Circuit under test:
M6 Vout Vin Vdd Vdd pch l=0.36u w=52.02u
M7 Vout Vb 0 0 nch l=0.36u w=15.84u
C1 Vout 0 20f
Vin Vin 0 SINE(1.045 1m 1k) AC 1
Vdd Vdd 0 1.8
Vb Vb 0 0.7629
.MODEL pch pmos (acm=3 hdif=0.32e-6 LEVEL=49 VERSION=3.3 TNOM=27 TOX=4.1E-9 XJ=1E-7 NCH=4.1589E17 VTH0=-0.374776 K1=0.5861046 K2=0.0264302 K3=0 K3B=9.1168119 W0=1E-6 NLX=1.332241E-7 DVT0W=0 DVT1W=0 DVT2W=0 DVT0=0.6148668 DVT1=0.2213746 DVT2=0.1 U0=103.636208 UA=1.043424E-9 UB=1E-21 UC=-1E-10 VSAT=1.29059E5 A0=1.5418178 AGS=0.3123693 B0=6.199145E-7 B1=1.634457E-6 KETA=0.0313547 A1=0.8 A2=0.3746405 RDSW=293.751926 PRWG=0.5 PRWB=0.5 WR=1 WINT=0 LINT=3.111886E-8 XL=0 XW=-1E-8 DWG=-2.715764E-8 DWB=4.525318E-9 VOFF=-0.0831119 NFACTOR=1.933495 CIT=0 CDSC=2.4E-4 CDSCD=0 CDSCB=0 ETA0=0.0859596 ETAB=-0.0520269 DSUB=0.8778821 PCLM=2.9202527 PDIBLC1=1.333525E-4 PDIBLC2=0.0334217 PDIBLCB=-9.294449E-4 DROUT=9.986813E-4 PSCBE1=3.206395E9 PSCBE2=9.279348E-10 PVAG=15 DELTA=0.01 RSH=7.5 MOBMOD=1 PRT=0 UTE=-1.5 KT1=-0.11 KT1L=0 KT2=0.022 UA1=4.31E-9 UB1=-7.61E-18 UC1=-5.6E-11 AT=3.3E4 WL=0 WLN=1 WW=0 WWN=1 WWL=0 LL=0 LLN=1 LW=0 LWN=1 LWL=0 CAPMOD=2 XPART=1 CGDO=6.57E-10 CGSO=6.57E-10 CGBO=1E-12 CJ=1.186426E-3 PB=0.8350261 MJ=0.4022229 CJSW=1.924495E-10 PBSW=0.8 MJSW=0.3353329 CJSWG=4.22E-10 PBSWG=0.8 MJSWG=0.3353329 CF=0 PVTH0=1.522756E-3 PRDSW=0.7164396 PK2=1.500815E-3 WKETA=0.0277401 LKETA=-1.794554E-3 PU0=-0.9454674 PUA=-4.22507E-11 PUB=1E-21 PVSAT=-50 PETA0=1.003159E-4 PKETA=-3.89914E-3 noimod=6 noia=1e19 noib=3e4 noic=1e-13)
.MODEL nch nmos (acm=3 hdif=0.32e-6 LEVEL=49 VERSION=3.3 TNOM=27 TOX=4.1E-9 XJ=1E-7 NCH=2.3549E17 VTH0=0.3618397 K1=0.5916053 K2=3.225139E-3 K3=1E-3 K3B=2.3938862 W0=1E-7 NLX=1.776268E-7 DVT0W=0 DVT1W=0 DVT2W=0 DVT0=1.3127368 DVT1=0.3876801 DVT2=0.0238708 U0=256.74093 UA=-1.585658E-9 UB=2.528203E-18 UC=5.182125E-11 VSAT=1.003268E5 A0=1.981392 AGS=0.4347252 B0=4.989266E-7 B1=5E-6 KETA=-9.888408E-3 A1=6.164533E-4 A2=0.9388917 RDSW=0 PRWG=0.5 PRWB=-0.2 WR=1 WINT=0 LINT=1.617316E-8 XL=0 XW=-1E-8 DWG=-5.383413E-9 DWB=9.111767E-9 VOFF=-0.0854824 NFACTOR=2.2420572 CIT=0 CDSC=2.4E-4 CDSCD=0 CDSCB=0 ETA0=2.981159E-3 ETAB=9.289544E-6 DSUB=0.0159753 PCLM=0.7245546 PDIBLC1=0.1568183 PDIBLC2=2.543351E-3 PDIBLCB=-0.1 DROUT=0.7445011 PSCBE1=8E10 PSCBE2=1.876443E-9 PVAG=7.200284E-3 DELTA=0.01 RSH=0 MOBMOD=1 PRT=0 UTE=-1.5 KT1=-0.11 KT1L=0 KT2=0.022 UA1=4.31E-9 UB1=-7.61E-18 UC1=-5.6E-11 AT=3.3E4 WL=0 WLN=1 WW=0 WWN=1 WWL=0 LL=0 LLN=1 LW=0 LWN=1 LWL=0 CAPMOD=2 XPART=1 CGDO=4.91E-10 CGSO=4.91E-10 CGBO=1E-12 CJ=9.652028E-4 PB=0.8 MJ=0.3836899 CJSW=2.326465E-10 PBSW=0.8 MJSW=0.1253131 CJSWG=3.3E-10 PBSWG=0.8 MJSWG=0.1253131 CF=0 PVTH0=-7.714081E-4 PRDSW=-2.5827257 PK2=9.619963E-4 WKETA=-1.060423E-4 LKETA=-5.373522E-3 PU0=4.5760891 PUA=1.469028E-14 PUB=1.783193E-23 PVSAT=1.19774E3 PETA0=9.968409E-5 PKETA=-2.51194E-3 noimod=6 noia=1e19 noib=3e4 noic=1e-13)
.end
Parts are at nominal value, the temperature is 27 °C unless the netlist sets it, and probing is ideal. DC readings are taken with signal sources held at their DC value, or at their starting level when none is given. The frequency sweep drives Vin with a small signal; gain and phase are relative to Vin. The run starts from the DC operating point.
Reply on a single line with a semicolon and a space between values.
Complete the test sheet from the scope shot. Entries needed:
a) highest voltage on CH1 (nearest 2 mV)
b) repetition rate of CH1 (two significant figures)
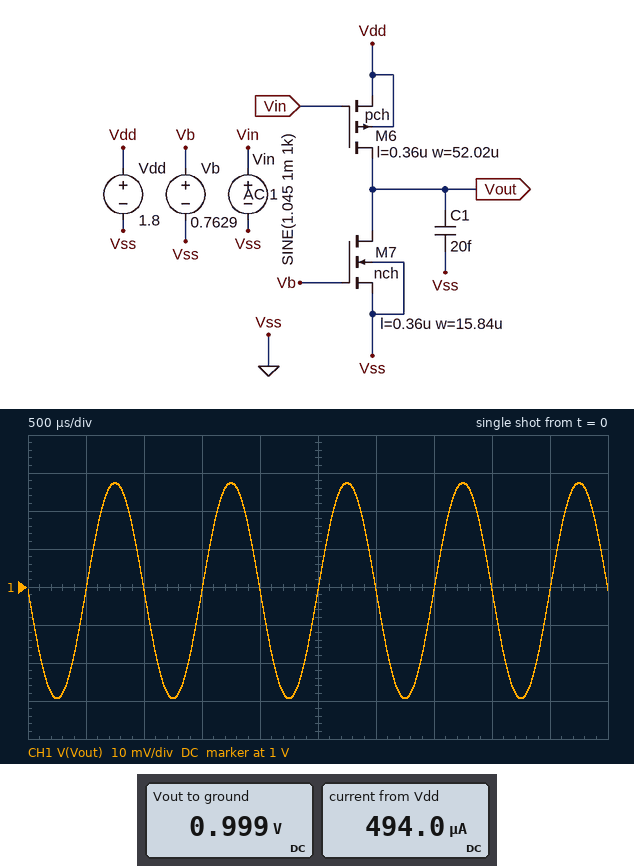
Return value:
1.028 V; 1.0 kHz
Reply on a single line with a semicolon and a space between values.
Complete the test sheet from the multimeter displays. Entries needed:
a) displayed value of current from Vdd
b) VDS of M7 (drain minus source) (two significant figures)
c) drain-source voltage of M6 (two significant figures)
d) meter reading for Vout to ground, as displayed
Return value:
494.0 µA; 1.0 V; -800 mV; 0.999 V
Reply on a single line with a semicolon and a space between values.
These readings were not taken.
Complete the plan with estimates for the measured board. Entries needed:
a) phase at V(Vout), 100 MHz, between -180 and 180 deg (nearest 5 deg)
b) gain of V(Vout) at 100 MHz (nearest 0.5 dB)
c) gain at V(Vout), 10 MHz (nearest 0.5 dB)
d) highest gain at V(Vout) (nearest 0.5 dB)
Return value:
140 deg; 27.0 dB; 29.0 dB; 29.0 dB
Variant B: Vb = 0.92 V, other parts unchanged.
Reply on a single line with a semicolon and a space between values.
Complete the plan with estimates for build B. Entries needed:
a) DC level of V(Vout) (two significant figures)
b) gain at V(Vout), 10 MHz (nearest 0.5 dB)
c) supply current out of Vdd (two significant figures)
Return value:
110 mV; -1.5 dB; 540 µA
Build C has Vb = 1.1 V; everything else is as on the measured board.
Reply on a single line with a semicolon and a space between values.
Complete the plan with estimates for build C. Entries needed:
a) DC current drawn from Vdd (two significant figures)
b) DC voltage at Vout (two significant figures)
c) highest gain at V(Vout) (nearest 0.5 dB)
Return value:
540 µA; 71 mV; -6.5 dB
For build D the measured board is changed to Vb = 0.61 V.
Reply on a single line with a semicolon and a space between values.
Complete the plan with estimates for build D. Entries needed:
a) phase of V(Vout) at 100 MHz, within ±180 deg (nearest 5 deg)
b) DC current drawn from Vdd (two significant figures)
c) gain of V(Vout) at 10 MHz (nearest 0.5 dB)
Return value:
170 deg; 140 µA; -14.5 dB
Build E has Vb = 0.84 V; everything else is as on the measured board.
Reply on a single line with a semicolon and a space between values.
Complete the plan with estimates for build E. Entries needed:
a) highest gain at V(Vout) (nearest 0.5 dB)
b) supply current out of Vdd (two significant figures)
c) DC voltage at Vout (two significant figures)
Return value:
4.0 dB; 540 µA; 160 mV
